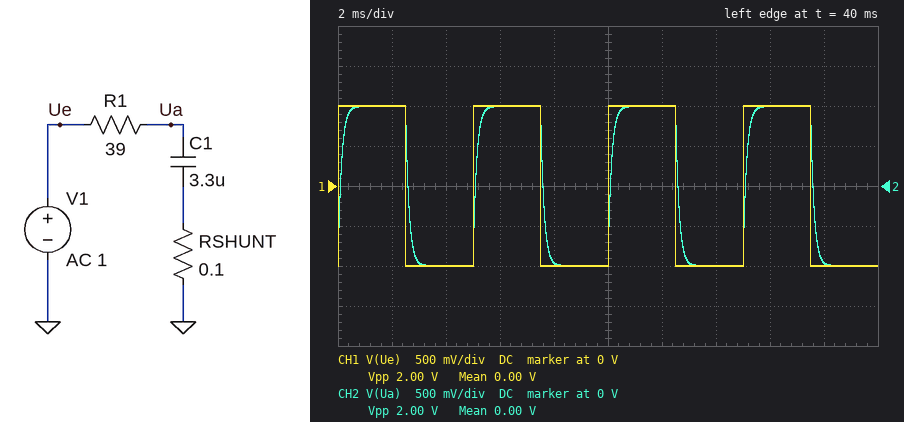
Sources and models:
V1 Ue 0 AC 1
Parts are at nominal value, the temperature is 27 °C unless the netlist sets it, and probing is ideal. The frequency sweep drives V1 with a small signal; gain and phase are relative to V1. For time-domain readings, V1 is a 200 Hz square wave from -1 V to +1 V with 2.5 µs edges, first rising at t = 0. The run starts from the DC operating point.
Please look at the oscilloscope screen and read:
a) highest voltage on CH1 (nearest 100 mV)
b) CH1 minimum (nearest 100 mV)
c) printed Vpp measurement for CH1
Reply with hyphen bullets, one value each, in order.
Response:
- 1.0 V
- -1.0 V
- 2.00 V
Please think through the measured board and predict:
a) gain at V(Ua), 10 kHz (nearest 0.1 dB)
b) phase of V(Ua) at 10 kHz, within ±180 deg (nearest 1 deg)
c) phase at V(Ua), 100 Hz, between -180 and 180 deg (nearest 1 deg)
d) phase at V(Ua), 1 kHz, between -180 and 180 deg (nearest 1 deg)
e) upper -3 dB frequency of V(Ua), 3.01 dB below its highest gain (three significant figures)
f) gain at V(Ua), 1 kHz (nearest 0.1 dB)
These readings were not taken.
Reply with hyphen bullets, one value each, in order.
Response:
- -18.2 dB
- -82 deg
- -5 deg
- -39 deg
- 1.23 kHz
- -2.2 dB
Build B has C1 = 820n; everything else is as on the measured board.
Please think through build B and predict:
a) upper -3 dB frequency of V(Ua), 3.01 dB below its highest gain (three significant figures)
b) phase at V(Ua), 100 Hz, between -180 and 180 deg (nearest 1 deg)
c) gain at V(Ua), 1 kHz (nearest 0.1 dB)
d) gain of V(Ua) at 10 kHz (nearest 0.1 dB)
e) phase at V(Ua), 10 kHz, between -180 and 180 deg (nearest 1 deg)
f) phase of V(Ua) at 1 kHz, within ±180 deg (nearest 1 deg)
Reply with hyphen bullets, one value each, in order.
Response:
- 4.96 kHz
- -1 deg
- -0.2 dB
- -7.0 dB
- -63 deg
- -11 deg
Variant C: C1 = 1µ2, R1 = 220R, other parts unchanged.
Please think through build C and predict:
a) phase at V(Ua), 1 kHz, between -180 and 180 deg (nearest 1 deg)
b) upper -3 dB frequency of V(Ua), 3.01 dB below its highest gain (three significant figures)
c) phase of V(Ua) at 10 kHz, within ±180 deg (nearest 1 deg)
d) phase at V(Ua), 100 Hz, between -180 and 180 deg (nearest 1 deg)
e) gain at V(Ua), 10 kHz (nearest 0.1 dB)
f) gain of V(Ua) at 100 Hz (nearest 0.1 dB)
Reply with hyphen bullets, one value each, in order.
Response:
- -59 deg
- 603 Hz
- -86 deg
- -9 deg
- -24.4 dB
- -0.1 dB
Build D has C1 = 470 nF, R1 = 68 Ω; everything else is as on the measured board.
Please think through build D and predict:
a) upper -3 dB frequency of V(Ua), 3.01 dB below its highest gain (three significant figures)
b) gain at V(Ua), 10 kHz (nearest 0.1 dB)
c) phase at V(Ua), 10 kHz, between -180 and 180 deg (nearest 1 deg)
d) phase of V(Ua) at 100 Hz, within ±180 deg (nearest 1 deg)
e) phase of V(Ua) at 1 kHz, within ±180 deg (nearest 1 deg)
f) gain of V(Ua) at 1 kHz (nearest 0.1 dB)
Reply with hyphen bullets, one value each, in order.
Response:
- 4.97 kHz
- -7.0 dB
- -63 deg
- -1 deg
- -11 deg
- -0.2 dB
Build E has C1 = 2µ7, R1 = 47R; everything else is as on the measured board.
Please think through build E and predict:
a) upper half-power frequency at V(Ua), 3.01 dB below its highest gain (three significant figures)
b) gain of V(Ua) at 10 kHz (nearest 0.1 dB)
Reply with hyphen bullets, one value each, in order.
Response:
- 1.25 kHz
- -18.1 dB
